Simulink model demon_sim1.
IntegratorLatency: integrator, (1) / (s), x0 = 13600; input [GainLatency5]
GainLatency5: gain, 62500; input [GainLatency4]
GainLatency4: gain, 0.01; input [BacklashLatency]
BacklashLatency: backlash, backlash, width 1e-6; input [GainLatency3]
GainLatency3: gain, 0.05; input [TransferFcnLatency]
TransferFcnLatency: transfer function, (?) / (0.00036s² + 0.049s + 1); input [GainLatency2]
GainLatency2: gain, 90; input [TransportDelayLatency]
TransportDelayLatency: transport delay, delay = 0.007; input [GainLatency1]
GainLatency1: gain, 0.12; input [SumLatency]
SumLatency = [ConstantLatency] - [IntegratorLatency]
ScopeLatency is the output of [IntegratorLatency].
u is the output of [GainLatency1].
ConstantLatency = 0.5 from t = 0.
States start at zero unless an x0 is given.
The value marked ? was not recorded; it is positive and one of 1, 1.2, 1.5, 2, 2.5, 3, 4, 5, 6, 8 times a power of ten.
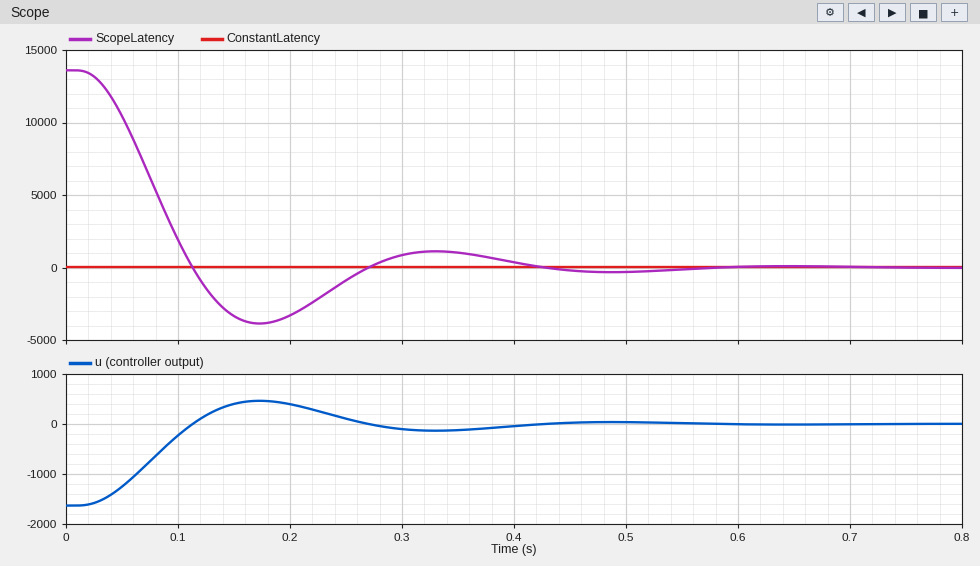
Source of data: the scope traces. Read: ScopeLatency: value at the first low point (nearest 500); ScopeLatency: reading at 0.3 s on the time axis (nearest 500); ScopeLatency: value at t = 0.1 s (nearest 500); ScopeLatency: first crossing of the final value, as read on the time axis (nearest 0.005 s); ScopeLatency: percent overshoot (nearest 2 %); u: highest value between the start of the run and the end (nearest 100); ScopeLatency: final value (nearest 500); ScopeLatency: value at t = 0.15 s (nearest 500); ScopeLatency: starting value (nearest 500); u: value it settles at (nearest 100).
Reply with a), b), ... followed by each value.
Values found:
a) -4000
b) 1000
c) 2000
d) 0.115 s
e) 28 %
f) 500
g) 0
h) -3500
i) 13500
j) 0
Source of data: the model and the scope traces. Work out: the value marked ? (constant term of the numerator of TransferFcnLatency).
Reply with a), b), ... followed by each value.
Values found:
a) 0.06
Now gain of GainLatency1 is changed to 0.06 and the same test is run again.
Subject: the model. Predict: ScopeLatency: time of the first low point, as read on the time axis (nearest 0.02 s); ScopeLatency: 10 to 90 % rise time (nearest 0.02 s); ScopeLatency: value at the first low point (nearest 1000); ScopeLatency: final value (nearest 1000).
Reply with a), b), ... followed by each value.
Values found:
a) 0.28 s
b) 0.12 s
c) -1000
d) 0
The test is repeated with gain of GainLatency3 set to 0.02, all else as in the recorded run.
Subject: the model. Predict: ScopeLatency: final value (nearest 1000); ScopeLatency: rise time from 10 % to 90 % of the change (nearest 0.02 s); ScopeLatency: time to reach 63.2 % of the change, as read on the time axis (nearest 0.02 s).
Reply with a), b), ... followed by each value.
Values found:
a) 0
b) 0.16 s
c) 0.14 s
